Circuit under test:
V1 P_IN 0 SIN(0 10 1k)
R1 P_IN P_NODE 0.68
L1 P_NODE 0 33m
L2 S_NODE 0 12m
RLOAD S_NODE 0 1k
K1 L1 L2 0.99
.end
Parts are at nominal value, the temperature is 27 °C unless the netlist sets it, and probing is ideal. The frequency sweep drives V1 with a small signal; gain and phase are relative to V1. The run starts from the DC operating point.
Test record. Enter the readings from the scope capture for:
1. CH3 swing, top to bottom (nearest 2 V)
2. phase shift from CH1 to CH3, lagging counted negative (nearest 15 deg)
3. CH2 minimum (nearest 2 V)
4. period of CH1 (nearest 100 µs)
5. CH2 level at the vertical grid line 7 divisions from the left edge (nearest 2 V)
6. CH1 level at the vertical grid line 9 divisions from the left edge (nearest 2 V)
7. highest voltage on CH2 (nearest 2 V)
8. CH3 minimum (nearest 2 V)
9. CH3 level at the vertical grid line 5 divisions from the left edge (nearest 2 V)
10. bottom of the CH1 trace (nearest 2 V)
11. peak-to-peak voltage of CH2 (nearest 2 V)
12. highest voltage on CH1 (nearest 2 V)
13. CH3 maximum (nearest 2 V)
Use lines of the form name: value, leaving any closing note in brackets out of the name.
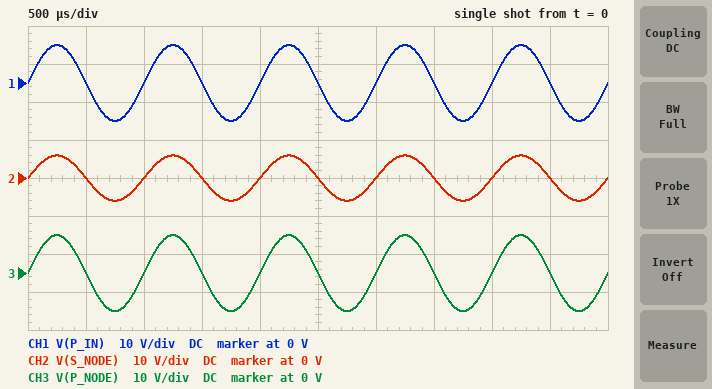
CH3 swing, top to bottom: 20 V
phase shift from CH1 to CH3, lagging counted negative: 0 deg
CH2 minimum: -6 V
period of CH1: 1.0 ms
CH2 level at the vertical grid line 7 divisions from the left edge: 0 V
CH1 level at the vertical grid line 9 divisions from the left edge: 0 V
highest voltage on CH2: 6 V
CH3 minimum: -10 V
CH3 level at the vertical grid line 5 divisions from the left edge: 0 V
bottom of the CH1 trace: -10 V
peak-to-peak voltage of CH2: 12 V
highest voltage on CH1: 10 V
CH3 maximum: 10 V
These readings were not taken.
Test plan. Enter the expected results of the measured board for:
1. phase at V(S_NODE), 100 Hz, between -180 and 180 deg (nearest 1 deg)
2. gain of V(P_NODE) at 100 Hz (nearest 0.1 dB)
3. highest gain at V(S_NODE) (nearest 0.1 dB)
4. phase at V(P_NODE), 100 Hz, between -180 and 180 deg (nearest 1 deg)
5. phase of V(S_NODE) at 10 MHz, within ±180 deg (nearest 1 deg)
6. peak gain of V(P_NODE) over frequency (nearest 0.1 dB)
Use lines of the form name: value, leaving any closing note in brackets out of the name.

phase at V(S_NODE), 100 Hz, between -180 and 180 deg: 2 deg
gain of V(P_NODE) at 100 Hz: 0 dB
highest gain at V(S_NODE): -4.5 dB
phase at V(P_NODE), 100 Hz, between -180 and 180 deg: 2 deg
phase of V(S_NODE) at 10 MHz, within ±180 deg: -86 deg
peak gain of V(P_NODE) over frequency: 0 dB
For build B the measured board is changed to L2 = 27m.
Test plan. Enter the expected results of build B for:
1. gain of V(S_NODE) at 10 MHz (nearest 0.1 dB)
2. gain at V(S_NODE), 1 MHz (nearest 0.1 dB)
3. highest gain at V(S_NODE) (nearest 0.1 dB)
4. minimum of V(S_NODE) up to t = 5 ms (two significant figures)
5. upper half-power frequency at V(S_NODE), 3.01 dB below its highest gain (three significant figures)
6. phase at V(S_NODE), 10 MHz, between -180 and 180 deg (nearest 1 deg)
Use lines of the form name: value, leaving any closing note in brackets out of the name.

gain of V(S_NODE) at 10 MHz: -31.5 dB
gain at V(S_NODE), 1 MHz: -11.9 dB
highest gain at V(S_NODE): -1.0 dB
minimum of V(S_NODE) up to t = 5 ms: -9.0 V
upper half-power frequency at V(S_NODE), 3.01 dB below its highest gain: 296 kHz
phase at V(S_NODE), 10 MHz, between -180 and 180 deg: -88 deg
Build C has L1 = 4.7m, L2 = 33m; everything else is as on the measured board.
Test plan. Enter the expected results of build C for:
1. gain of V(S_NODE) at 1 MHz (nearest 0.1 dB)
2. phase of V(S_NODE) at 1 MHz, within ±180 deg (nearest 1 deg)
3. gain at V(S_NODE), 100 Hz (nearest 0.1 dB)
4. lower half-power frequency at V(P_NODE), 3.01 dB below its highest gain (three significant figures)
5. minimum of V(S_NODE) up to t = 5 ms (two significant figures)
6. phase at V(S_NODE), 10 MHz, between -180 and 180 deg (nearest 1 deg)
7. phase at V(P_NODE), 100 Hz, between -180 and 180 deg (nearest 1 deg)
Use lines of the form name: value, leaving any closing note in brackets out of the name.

gain of V(S_NODE) at 1 MHz: -4.2 dB
phase of V(S_NODE) at 1 MHz, within ±180 deg: -76 deg
gain at V(S_NODE), 100 Hz: 8.1 dB
lower half-power frequency at V(P_NODE), 3.01 dB below its highest gain: 23.1 Hz
minimum of V(S_NODE) up to t = 5 ms: -27 V
phase at V(S_NODE), 10 MHz, between -180 and 180 deg: -89 deg
phase at V(P_NODE), 100 Hz, between -180 and 180 deg: 13 deg
